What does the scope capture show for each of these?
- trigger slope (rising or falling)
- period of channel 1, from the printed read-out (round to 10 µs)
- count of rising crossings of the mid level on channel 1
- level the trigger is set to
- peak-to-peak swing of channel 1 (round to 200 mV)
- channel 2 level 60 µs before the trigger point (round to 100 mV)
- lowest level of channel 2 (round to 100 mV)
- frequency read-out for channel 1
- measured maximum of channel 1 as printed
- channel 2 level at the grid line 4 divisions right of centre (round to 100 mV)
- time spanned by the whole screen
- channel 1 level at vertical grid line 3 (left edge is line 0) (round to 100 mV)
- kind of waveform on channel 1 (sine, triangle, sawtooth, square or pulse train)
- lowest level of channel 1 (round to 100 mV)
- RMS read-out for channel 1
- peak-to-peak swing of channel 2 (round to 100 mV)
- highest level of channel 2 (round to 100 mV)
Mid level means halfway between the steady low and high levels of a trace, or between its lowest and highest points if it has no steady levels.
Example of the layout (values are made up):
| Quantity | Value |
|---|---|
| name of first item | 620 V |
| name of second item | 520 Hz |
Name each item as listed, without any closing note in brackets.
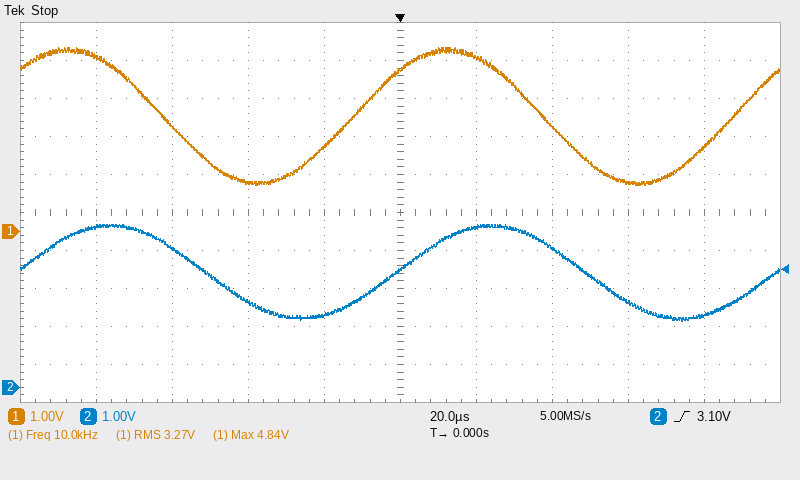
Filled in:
| Quantity | Value |
|---|---|
| trigger slope | rising |
| period of channel 1, from the printed read-out | 100 µs |
| count of rising crossings of the mid level on channel 1 | 2 |
| level the trigger is set to | 3.10 V |
| peak-to-peak swing of channel 1 | 3.6 V |
| channel 2 level 60 µs before the trigger point | 3.6 V |
| lowest level of channel 2 | 1.7 V |
| frequency read-out for channel 1 | 10.0 kHz |
| measured maximum of channel 1 as printed | 4.84 V |
| channel 2 level at the grid line 4 divisions right of centre | 1.9 V |
| time spanned by the whole screen | 200 µs |
| channel 1 level at vertical grid line 3 (left edge is line 0) | 1.3 V |
| kind of waveform on channel 1 | sine |
| lowest level of channel 1 | 1.2 V |
| RMS read-out for channel 1 | 3.27 V |
| peak-to-peak swing of channel 2 | 2.6 V |
| highest level of channel 2 | 4.3 V |
